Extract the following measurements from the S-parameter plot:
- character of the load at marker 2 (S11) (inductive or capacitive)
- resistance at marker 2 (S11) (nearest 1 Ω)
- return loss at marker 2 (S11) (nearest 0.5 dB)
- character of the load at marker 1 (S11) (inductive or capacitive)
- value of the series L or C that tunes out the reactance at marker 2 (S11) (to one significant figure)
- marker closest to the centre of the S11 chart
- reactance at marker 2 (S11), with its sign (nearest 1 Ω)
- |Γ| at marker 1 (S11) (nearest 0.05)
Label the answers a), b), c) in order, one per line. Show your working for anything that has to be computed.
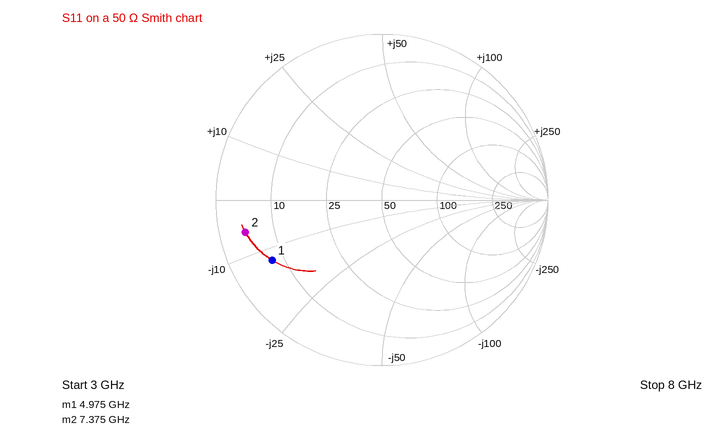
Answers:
a) capacitive
b) 4 Ω
c) 1.5 dB
d) capacitive
e) L = 6 Ω/(2π × 7.375 GHz) ≈ 129 pH, so 100 pH to one significant figure
f) marker 1
g) -6 Ω
h) 0.75
